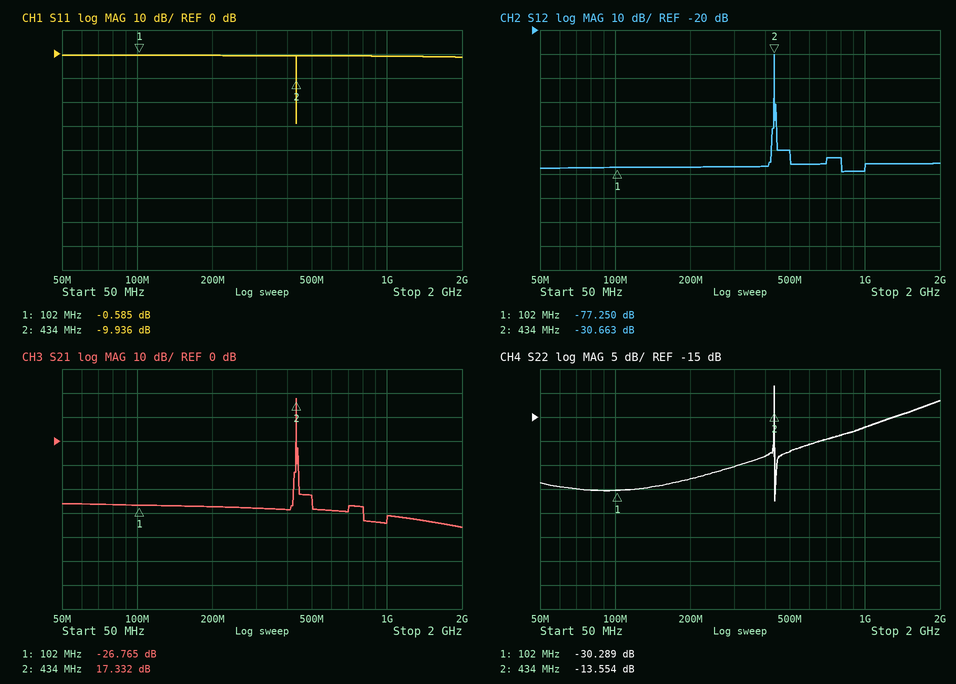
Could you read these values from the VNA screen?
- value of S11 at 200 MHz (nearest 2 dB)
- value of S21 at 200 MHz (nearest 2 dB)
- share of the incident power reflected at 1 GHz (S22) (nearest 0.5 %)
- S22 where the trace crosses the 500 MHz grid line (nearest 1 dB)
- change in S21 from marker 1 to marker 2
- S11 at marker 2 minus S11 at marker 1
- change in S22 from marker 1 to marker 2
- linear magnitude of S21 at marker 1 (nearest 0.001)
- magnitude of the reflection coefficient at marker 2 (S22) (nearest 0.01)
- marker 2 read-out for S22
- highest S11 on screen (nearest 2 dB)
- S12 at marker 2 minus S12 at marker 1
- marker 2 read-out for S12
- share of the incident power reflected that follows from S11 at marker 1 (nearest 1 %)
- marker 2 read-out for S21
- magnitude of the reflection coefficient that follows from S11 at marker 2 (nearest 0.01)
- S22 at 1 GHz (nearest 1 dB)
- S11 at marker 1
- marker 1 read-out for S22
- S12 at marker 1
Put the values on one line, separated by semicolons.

0 dB; -28 dB; 2.0 %; -22 dB; 44.097 dB; -9.351 dB; 16.735 dB; 0.046; 0.21; -13.554 dB; 0 dB; 46.587 dB; -30.663 dB; 87 %; 17.332 dB; 0.32; -17 dB; -0.585 dB; -30.289 dB; -77.250 dB
